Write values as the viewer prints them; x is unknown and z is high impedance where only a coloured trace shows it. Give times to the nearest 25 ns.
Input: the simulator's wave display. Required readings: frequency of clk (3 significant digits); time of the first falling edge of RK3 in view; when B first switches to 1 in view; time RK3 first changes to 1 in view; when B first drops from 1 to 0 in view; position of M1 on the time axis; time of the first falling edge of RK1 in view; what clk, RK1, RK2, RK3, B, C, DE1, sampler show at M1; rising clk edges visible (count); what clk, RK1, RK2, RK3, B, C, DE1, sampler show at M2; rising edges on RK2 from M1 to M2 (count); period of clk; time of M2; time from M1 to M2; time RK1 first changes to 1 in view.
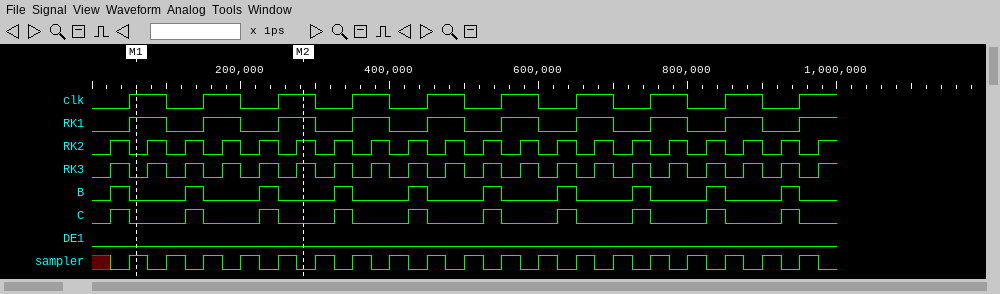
10.0 MHz
50 ns
25 ns
25 ns
50 ns
50 ns
100 ns
clk=1, RK1=1, RK2=0, RK3=0, B=0, C=0, DE1=0, sampler=1
10
clk=1, RK1=1, RK2=1, RK3=1, B=0, C=0, DE1=0, sampler=0
5
100 ns
275 ns
225 ns
50 ns
